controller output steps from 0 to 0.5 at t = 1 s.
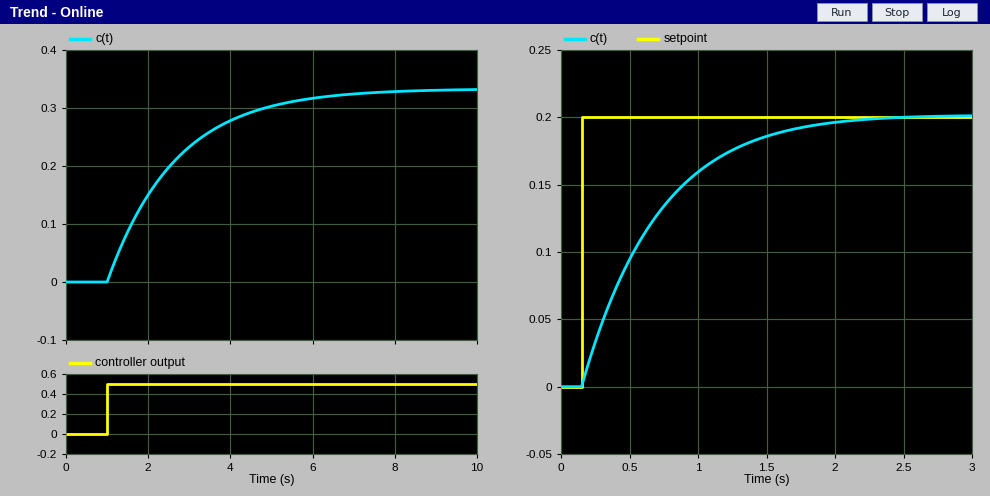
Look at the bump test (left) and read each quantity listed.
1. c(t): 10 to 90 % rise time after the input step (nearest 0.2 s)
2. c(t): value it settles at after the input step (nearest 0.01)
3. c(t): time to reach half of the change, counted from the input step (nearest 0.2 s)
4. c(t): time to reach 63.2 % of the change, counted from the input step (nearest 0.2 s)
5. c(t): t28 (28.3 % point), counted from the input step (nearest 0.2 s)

3.6 s
0.33
1.2 s
1.6 s
0.6 s
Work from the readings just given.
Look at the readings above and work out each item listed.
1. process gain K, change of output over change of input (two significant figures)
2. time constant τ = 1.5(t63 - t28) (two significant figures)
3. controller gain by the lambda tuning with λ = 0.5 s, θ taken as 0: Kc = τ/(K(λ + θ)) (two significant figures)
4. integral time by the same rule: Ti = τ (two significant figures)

0.66
1.5 s
4.5
1.5 s
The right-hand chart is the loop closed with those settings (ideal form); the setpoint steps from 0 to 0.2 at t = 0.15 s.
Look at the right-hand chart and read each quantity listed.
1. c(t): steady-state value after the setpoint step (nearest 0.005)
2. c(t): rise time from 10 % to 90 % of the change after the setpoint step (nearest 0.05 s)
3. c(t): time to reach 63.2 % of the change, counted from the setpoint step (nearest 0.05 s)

0.200
1.15 s
0.55 s
